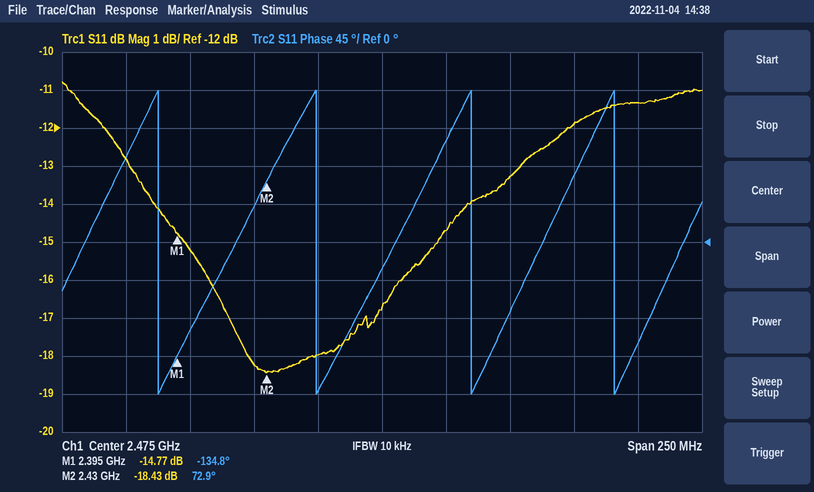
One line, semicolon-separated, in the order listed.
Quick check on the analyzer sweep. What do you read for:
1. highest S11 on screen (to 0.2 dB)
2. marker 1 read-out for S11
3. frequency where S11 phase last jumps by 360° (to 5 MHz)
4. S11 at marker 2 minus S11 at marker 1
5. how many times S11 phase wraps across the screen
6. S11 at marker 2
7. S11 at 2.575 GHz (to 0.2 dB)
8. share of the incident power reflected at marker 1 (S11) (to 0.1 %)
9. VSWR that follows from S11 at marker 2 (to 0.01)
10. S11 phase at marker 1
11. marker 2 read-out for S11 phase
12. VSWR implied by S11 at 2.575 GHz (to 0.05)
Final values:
-10.8 dB; -14.77 dB; 2.565 GHz; -3.66 dB; 4; -18.43 dB; -11.4 dB; 3.3 %; 1.27; -134.8°; 72.9°; 1.75
